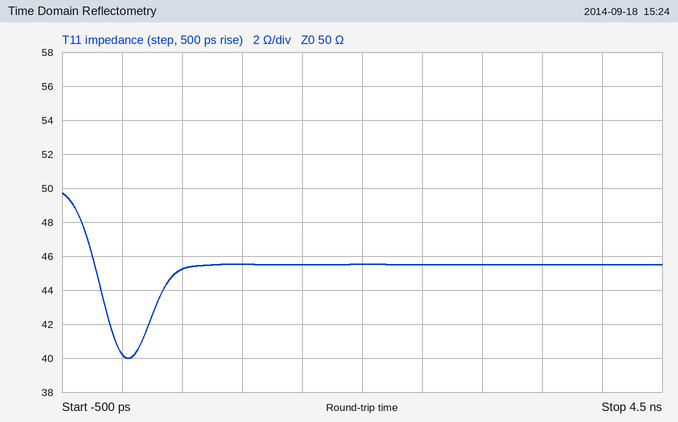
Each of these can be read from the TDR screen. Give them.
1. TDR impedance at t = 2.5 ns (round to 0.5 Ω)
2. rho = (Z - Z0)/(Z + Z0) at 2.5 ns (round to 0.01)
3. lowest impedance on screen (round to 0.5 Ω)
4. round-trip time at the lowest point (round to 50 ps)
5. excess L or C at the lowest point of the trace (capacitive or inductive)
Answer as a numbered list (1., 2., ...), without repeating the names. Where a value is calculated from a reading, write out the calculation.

1. 45.5 Ω
2. (45.5 − 50)/(45.5 + 50) ≈ -0.05
3. 40.0 Ω
4. 50 ps
5. capacitive
